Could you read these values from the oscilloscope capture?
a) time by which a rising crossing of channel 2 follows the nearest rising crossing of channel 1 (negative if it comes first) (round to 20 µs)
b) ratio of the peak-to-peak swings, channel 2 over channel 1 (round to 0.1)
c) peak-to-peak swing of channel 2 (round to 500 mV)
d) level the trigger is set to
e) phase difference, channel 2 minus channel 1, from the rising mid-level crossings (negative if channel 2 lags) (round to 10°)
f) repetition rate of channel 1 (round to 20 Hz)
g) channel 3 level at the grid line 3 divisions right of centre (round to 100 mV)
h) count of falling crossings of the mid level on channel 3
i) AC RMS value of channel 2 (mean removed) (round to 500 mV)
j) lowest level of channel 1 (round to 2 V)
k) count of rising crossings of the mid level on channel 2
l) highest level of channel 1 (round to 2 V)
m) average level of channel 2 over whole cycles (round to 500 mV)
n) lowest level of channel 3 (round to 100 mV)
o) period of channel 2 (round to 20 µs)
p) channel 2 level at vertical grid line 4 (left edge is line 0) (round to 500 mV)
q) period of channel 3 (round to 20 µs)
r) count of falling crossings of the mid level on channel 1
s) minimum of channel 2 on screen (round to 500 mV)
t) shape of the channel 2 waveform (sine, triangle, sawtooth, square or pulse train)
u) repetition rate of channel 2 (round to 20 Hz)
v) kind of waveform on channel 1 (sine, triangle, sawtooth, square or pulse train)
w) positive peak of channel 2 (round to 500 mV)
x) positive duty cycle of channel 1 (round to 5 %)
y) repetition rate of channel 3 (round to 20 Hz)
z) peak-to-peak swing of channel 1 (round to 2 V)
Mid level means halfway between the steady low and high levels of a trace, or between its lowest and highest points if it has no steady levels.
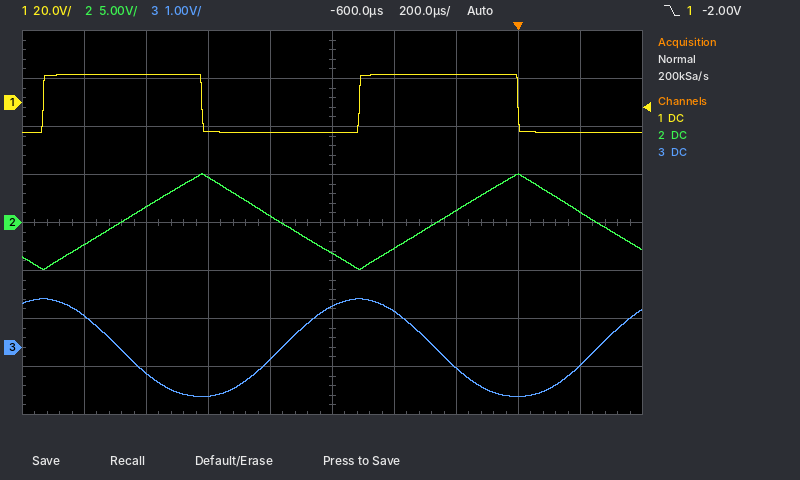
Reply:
+260 µs
0.4
10.0 V
-2.00 V
-90°
980 Hz
-1.0 V
2
3.0 V
-12 V
2
12 V
0.0 V
-1.0 V
1.02 ms
500 mV
1.02 ms
2
-5.0 V
triangle
980 Hz
square
5.0 V
50 %
980 Hz
24 V
